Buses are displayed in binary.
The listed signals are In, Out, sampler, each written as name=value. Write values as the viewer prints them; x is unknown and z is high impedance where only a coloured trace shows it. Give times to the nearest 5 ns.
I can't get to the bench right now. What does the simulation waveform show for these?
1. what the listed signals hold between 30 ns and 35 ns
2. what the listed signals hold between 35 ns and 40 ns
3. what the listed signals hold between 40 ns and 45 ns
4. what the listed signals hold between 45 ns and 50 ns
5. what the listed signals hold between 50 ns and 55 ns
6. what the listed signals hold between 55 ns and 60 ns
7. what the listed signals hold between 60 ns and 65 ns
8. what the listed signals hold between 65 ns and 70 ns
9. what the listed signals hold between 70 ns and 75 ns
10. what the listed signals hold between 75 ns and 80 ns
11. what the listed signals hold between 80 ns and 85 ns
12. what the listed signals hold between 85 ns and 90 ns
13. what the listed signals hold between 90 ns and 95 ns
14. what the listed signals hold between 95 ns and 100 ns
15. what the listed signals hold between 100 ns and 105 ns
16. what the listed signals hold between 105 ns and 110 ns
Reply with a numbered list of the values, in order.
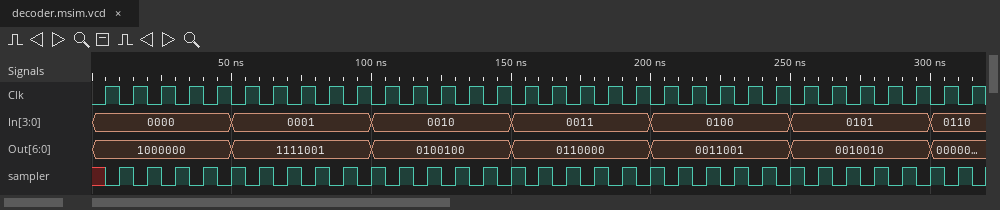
1. In=0000, Out=1000000, sampler=1
2. In=0000, Out=1000000, sampler=0
3. In=0000, Out=1000000, sampler=1
4. In=0000, Out=1000000, sampler=0
5. In=0001, Out=1111001, sampler=1
6. In=0001, Out=1111001, sampler=0
7. In=0001, Out=1111001, sampler=1
8. In=0001, Out=1111001, sampler=0
9. In=0001, Out=1111001, sampler=1
10. In=0001, Out=1111001, sampler=0
11. In=0001, Out=1111001, sampler=1
12. In=0001, Out=1111001, sampler=0
13. In=0001, Out=1111001, sampler=1
14. In=0001, Out=1111001, sampler=0
15. In=0010, Out=0100100, sampler=1
16. In=0010, Out=0100100, sampler=0
